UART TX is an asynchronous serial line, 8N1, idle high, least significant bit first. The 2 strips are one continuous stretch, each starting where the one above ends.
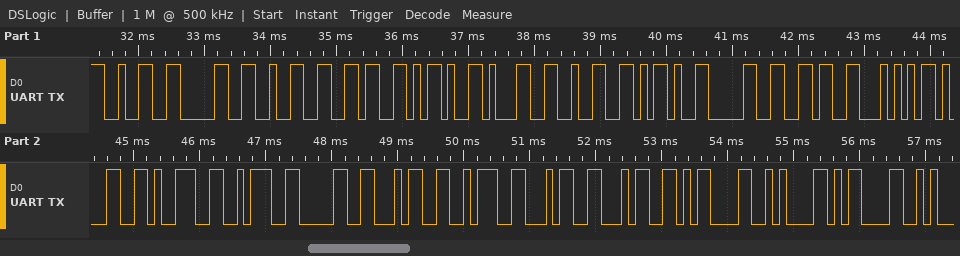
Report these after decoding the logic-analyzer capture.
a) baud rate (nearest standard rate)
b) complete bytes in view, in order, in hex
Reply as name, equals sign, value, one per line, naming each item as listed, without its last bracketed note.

baud rate = 9600 baud
complete bytes in view, in order, in hex = 0x32 0x30 0x32 0x36 0x2D 0x31 0x32 0x2D 0x30 0x36 0x54 0x31 0x39 0x3A 0x30 0x34 0x3A 0x34 0x34 0x0D 0x0A 0x0D
